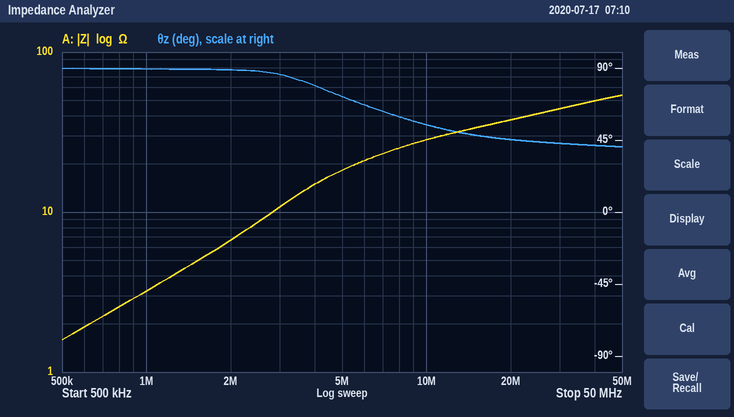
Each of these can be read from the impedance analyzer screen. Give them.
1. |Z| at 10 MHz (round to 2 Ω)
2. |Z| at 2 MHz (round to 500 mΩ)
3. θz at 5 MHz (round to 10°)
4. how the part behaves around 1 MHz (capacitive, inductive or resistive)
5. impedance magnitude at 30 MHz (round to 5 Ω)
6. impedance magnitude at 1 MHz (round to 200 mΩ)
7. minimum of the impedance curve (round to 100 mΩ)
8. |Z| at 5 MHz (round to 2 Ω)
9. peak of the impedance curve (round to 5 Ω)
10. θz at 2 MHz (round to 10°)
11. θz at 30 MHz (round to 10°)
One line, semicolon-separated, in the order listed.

28 Ω; 6.5 Ω; 70°; inductive; 45 Ω; 3.2 Ω; 1.6 Ω; 18 Ω; 55 Ω; 90°; 40°
